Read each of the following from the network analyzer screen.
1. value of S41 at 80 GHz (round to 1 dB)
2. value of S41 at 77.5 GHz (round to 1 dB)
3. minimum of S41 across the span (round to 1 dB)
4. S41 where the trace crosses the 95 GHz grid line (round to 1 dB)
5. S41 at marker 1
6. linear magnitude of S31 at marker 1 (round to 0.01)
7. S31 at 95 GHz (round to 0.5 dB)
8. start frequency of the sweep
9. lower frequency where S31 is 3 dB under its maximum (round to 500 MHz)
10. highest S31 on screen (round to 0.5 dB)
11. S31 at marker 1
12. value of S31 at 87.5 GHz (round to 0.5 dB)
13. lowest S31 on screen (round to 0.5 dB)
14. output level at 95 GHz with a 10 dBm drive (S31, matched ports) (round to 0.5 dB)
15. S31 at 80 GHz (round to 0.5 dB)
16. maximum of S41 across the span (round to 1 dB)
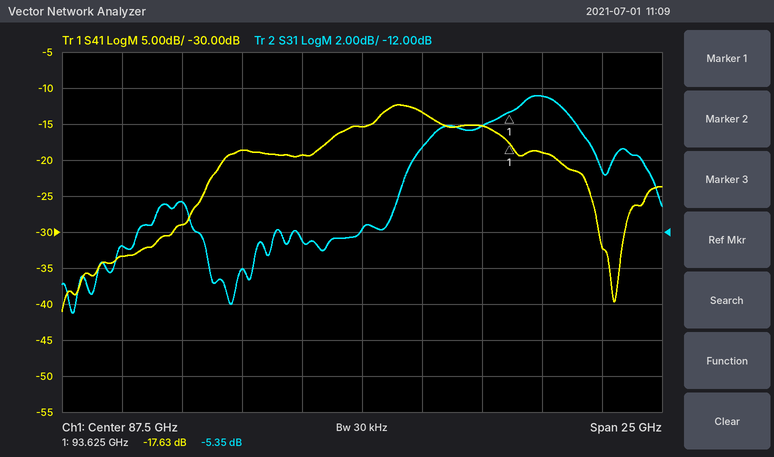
-29 dB
-33 dB
-41 dB
-19 dB
-17.63 dB
0.54
-4.5 dB
75 GHz
90.0 GHz
-4.5 dB
-5.35 dB
-12.0 dB
-16.5 dB
5.5 dBm
-10.5 dB
-12 dB
